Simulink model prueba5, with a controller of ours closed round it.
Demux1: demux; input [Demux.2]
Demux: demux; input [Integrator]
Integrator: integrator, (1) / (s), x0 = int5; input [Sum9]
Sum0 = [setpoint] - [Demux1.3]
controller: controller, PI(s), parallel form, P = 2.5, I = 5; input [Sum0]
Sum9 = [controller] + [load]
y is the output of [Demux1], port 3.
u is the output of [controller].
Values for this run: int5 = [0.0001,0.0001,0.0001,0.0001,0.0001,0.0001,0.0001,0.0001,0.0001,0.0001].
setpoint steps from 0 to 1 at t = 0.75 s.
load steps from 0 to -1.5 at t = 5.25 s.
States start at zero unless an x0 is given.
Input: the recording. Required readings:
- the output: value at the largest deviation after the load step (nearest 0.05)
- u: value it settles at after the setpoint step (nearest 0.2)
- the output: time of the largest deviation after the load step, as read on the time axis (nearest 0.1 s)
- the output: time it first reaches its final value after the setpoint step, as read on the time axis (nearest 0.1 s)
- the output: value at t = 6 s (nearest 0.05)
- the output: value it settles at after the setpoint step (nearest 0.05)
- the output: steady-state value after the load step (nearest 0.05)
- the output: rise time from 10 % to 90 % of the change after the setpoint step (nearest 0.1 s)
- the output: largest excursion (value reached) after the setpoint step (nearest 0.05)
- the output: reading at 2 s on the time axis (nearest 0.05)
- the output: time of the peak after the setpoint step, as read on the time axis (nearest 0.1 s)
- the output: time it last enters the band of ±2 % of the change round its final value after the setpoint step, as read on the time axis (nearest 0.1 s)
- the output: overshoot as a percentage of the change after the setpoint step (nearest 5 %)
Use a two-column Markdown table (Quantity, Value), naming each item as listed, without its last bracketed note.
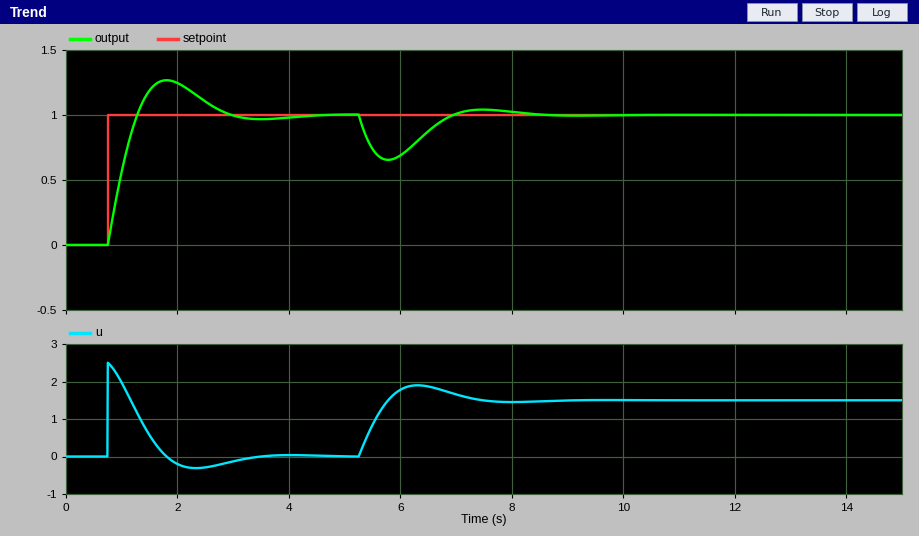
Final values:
| Quantity | Value |
|---|---|
| the output: value at the largest deviation after the load step | 0.65 |
| u: value it settles at after the setpoint step | 0.0 |
| the output: time of the largest deviation after the load step, as read on the time axis | 5.8 s |
| the output: time it first reaches its final value after the setpoint step, as read on the time axis | 1.3 s |
| the output: value at t = 6 s | 0.70 |
| the output: value it settles at after the setpoint step | 1.00 |
| the output: steady-state value after the load step | 1.00 |
| the output: rise time from 10 % to 90 % of the change after the setpoint step | 0.4 s |
| the output: largest excursion (value reached) after the setpoint step | 1.25 |
| the output: reading at 2 s on the time axis | 1.25 |
| the output: time of the peak after the setpoint step, as read on the time axis | 1.8 s |
| the output: time it last enters the band of ±2 % of the change round its final value after the setpoint step, as read on the time axis | 4.0 s |
| the output: overshoot as a percentage of the change after the setpoint step | 25 % |
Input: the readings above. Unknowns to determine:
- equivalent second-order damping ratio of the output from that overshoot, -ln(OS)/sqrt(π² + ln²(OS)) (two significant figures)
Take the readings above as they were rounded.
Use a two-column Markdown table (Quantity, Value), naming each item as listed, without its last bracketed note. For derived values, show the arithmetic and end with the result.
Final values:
| Quantity | Value |
|---|---|
| equivalent second-order damping ratio of the output from that overshoot, -ln(OS)/sqrt(π² + ln²(OS)) | ln(0.25) = -1.386; 1.386 / sqrt(9.870 + 1.922) = 0.40 |
